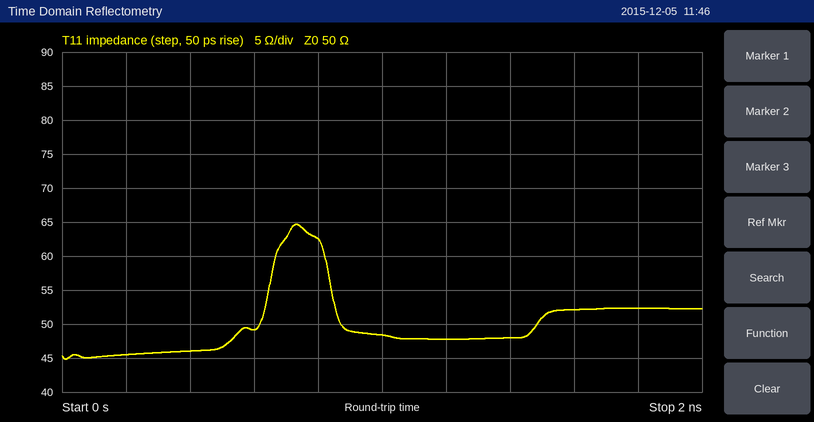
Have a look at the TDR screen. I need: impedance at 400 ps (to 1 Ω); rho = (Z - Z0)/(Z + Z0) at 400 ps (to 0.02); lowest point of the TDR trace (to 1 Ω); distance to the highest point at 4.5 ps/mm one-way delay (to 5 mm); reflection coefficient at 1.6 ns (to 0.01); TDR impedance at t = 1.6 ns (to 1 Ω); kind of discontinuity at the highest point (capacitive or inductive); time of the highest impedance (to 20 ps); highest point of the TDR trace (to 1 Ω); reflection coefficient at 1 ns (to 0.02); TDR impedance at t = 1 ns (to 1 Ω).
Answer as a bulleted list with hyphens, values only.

- 46 Ω
- -0.04
- 45 Ω
- 80 mm
- +0.02
- 52 Ω
- inductive
- 740 ps
- 65 Ω
- -0.02
- 48 Ω
